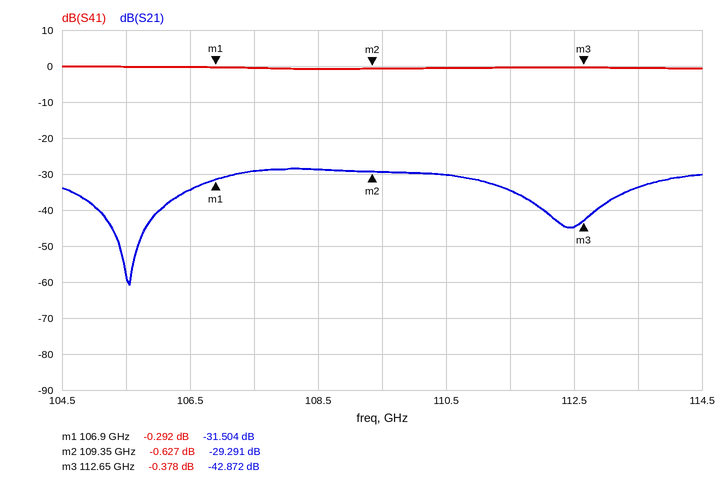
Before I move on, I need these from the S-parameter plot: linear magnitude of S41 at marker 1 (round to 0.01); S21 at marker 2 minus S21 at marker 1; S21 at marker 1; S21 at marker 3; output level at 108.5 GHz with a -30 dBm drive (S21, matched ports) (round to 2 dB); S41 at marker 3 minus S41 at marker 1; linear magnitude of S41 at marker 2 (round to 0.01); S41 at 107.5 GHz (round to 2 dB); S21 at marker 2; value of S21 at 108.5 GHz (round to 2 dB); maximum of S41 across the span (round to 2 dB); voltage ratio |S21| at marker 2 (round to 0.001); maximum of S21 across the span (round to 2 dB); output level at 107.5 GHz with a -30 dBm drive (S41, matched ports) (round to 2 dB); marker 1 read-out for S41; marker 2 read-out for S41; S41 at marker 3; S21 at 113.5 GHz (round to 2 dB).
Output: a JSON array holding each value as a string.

["0.97", "2.213 dB", "-31.504 dB", "-42.872 dB", "-58 dBm", "-0.086 dB", "0.93", "0 dB", "-29.291 dB", "-28 dB", "0 dB", "0.034", "-28 dB", "-30 dBm", "-0.292 dB", "-0.627 dB", "-0.378 dB", "-34 dB"]
